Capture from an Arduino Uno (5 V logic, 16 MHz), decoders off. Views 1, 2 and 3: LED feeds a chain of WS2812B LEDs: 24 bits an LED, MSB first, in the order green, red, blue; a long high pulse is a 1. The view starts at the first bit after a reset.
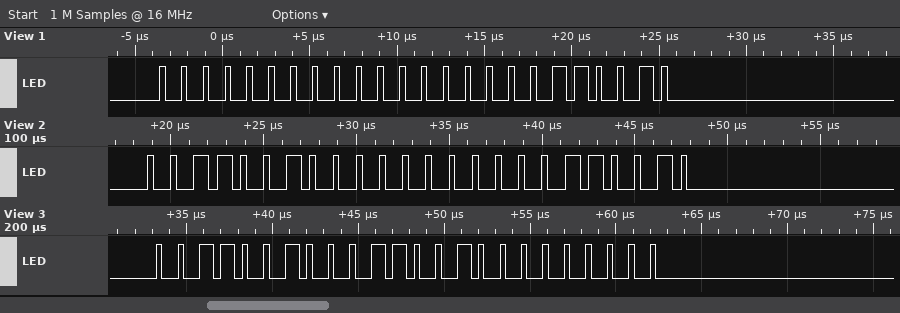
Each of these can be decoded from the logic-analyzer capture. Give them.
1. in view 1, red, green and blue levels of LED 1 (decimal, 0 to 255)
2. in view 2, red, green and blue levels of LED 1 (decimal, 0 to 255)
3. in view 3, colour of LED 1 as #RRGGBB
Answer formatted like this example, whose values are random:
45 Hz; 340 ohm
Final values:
0, 0, 50; 0, 50, 50; #323200
